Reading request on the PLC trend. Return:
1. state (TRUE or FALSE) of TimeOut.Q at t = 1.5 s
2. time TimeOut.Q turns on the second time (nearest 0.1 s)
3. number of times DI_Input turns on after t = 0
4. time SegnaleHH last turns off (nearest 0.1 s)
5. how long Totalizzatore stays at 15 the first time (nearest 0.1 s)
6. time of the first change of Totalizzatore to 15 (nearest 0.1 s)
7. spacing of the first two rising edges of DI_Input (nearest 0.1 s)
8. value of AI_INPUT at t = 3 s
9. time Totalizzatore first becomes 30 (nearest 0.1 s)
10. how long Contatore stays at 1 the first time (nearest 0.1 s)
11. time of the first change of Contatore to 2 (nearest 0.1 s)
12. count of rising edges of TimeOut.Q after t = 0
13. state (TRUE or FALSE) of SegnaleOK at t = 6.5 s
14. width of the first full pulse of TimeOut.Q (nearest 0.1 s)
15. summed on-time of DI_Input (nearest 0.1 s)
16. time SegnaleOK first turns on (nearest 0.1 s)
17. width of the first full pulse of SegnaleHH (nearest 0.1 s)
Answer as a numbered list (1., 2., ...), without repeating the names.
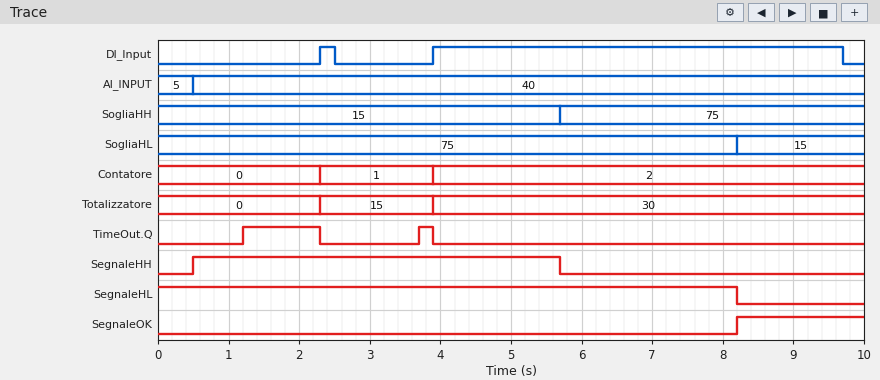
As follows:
1. TRUE
2. 3.7 s
3. 2
4. 5.7 s
5. 1.6 s
6. 2.3 s
7. 1.6 s
8. 40
9. 3.9 s
10. 1.6 s
11. 3.9 s
12. 2
13. FALSE
14. 1.1 s
15. 6.0 s
16. 8.2 s
17. 5.2 s
